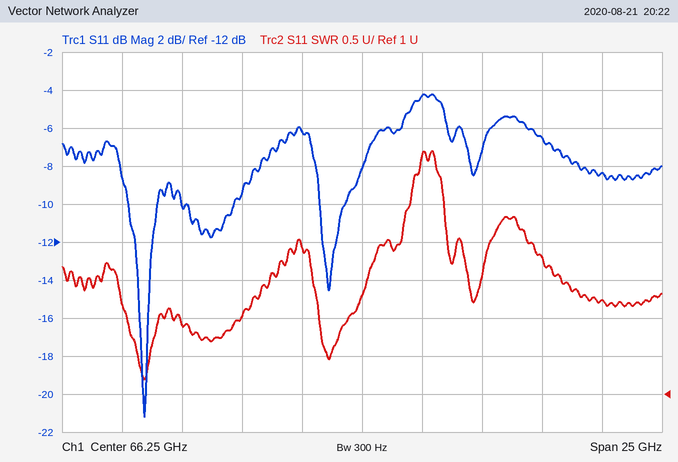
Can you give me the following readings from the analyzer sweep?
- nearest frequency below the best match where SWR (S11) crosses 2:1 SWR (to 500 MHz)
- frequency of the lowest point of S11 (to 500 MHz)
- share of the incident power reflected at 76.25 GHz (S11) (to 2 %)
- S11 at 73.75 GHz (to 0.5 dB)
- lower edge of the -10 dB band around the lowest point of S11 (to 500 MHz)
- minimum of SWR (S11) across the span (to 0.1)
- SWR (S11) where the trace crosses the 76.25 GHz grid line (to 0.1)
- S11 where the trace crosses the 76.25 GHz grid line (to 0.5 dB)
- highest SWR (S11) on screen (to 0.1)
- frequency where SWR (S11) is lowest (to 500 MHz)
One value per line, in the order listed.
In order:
56.5 GHz
57.0 GHz
14 %
-6.5 dB
56.5 GHz
1.2
2.2
-8.5 dB
4.2
57.0 GHz
